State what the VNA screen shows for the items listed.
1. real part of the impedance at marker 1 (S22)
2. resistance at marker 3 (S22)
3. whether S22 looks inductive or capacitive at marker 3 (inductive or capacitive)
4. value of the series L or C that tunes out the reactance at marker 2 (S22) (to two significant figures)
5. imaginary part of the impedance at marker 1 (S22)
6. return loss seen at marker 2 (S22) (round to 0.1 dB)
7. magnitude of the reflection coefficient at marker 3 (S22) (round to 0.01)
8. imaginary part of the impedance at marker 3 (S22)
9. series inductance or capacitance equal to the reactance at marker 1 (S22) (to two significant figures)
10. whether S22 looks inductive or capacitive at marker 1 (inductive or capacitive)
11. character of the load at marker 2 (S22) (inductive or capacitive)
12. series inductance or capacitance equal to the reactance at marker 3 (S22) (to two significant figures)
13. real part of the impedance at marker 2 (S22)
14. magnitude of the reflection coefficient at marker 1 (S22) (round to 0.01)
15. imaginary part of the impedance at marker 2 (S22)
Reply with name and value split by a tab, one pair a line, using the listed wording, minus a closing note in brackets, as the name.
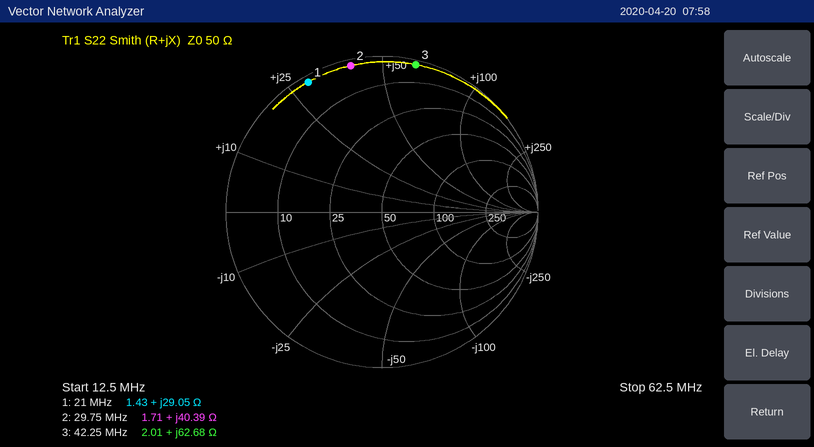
real part of the impedance at marker 1	1.43 Ω
resistance at marker 3	2.01 Ω
whether S22 looks inductive or capacitive at marker 3	inductive
value of the series L or C that tunes out the reactance at marker 2 (S22)	130 pF
imaginary part of the impedance at marker 1	+29.05 Ω
return loss seen at marker 2 (S22)	0.4 dB
magnitude of the reflection coefficient at marker 3 (S22)	0.97
imaginary part of the impedance at marker 3	+62.68 Ω
series inductance or capacitance equal to the reactance at marker 1 (S22)	220 nH
whether S22 looks inductive or capacitive at marker 1	inductive
character of the load at marker 2 (S22)	inductive
series inductance or capacitance equal to the reactance at marker 3 (S22)	240 nH
real part of the impedance at marker 2	1.71 Ω
magnitude of the reflection coefficient at marker 1 (S22)	0.96
imaginary part of the impedance at marker 2	+40.39 Ω
